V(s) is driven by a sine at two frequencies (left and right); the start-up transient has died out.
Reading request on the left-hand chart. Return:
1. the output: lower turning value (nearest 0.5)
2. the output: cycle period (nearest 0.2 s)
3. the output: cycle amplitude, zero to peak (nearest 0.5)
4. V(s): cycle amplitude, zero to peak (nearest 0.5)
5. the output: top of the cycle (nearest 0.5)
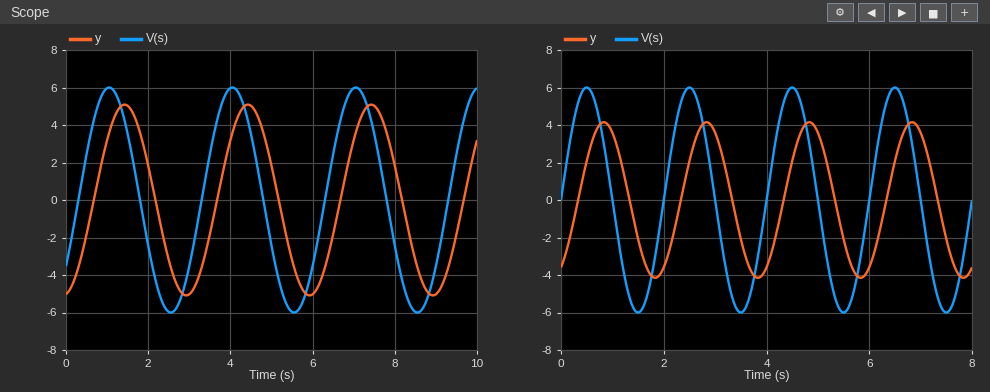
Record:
-5.0
3.0 s
5.0
6.0
5.0
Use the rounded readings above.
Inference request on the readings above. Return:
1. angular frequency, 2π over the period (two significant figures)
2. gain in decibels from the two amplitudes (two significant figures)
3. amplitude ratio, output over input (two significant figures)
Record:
2.1 rad/s
-1.6 dB
0.83
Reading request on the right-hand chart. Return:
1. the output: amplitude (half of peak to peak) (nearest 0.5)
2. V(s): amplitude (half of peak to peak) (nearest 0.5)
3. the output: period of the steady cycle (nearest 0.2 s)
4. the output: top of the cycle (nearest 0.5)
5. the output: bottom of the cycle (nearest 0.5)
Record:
4.0
6.0
2.0 s
4.0
-4.0
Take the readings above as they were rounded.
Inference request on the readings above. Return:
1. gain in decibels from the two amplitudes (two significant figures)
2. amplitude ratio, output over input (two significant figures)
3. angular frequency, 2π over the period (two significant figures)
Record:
-3.5 dB
0.67
3.1 rad/s
